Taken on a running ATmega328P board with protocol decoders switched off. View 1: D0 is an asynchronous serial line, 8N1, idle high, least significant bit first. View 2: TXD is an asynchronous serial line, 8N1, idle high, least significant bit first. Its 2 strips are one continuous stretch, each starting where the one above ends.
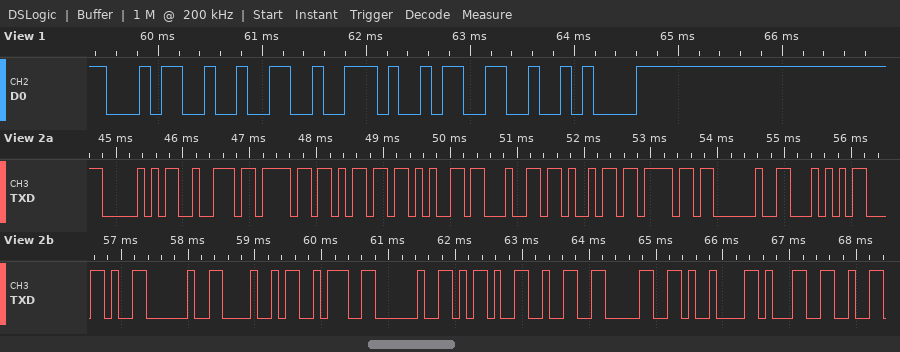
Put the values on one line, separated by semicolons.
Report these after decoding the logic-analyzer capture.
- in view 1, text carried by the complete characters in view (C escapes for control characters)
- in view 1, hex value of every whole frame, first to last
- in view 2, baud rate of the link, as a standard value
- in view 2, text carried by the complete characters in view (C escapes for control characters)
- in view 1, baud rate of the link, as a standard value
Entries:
"42.3\n"; 0x34 0x32 0x2E 0x33 0x0A; 9600 baud; "Promedio T, H: -20\t1"; 9600 baud
